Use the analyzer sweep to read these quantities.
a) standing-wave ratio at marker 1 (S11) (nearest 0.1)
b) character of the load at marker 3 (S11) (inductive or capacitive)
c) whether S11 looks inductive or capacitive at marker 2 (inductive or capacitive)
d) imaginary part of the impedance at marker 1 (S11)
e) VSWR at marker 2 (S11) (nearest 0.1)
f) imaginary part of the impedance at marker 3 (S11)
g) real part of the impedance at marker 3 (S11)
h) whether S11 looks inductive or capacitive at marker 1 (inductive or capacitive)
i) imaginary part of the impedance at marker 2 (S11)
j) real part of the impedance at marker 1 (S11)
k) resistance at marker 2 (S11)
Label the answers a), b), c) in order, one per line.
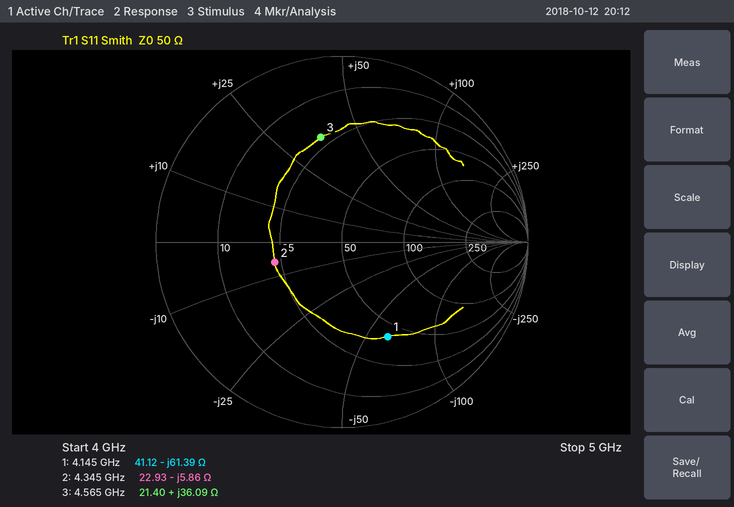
a) 3.6
b) inductive
c) capacitive
d) -61.39 Ω
e) 2.2
f) +36.09 Ω
g) 21.40 Ω
h) capacitive
i) -5.86 Ω
j) 41.12 Ω
k) 22.93 Ω
